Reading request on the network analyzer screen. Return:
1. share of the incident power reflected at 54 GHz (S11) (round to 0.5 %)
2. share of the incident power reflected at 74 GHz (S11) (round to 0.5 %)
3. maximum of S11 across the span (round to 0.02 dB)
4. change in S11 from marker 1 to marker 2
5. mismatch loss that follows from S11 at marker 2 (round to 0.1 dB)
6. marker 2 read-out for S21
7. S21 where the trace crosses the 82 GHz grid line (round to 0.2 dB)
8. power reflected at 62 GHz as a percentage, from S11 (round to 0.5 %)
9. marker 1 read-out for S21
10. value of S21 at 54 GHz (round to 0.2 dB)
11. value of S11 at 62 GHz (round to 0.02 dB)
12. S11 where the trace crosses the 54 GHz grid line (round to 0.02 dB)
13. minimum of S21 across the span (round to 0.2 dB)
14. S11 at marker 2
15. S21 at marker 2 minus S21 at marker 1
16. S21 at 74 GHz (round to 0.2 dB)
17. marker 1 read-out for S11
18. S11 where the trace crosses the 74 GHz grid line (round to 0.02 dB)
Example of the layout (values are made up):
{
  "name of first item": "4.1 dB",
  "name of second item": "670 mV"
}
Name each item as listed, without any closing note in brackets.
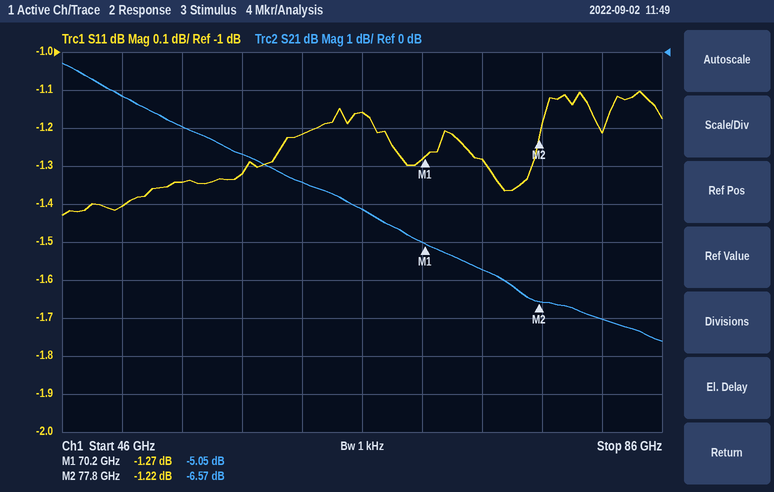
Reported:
{
  "share of the incident power reflected at 54 GHz (S11)": "73.5 %",
  "share of the incident power reflected at 74 GHz (S11)": "74.5 %",
  "maximum of S11 across the span": "-1.10 dB",
  "change in S11 from marker 1 to marker 2": "0.05 dB",
  "mismatch loss that follows from S11 at marker 2": "6.1 dB",
  "marker 2 read-out for S21": "-6.57 dB",
  "S21 where the trace crosses the 82 GHz grid line": "-7.0 dB",
  "power reflected at 62 GHz as a percentage, from S11": "75.5 %",
  "marker 1 read-out for S21": "-5.05 dB",
  "value of S21 at 54 GHz": "-2.0 dB",
  "value of S11 at 62 GHz": "-1.22 dB",
  "S11 where the trace crosses the 54 GHz grid line": "-1.34 dB",
  "minimum of S21 across the span": "-7.6 dB",
  "S11 at marker 2": "-1.22 dB",
  "S21 at marker 2 minus S21 at marker 1": "-1.52 dB",
  "S21 at 74 GHz": "-5.8 dB",
  "marker 1 read-out for S11": "-1.27 dB",
  "S11 where the trace crosses the 74 GHz grid line": "-1.28 dB"
}
